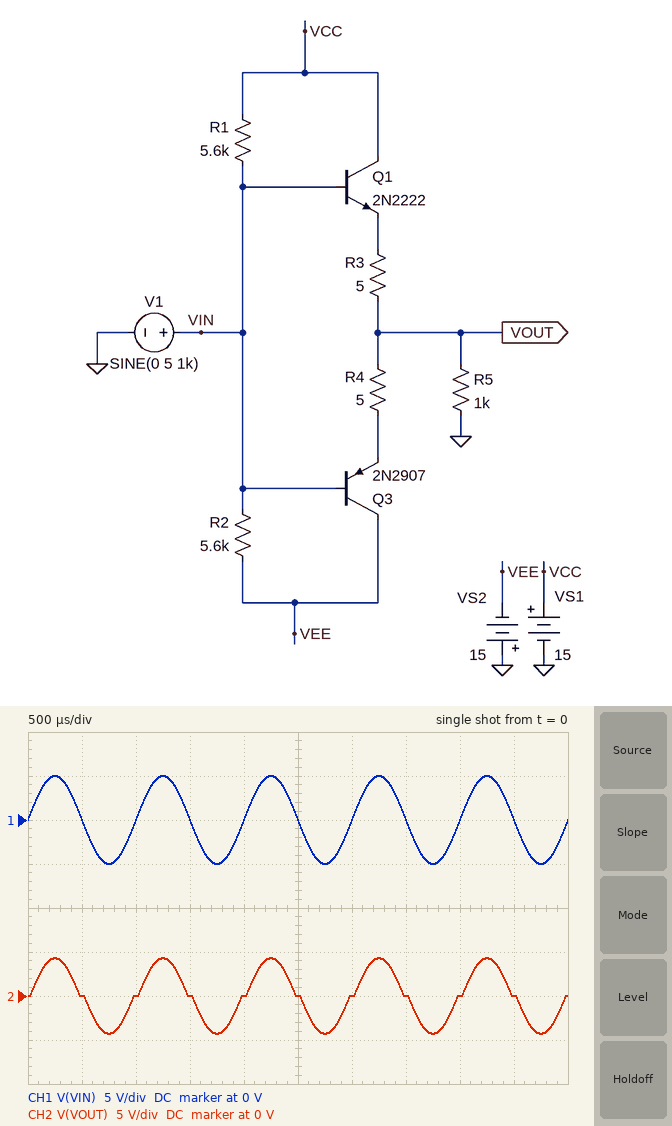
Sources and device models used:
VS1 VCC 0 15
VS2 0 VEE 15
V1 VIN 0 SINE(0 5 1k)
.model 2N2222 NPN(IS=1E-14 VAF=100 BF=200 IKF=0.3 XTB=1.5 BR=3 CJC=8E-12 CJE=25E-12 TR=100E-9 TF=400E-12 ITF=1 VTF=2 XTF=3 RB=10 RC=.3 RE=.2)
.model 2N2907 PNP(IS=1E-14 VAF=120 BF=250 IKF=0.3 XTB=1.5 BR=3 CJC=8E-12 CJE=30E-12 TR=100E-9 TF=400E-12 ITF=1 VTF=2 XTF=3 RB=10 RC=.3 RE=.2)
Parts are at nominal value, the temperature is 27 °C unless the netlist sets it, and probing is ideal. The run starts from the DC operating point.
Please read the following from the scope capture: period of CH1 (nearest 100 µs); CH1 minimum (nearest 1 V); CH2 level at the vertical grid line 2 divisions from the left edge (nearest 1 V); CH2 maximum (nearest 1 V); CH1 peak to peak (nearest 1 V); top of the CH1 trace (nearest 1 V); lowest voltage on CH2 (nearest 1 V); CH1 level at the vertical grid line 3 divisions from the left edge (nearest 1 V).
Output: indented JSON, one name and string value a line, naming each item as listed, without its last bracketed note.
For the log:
{
  "period of CH1": "1.0 ms",
  "CH1 minimum": "-5 V",
  "CH2 level at the vertical grid line 2 divisions from the left edge": "0 V",
  "CH2 maximum": "4 V",
  "CH1 peak to peak": "10 V",
  "top of the CH1 trace": "5 V",
  "lowest voltage on CH2": "-4 V",
  "CH1 level at the vertical grid line 3 divisions from the left edge": "0 V"
}
